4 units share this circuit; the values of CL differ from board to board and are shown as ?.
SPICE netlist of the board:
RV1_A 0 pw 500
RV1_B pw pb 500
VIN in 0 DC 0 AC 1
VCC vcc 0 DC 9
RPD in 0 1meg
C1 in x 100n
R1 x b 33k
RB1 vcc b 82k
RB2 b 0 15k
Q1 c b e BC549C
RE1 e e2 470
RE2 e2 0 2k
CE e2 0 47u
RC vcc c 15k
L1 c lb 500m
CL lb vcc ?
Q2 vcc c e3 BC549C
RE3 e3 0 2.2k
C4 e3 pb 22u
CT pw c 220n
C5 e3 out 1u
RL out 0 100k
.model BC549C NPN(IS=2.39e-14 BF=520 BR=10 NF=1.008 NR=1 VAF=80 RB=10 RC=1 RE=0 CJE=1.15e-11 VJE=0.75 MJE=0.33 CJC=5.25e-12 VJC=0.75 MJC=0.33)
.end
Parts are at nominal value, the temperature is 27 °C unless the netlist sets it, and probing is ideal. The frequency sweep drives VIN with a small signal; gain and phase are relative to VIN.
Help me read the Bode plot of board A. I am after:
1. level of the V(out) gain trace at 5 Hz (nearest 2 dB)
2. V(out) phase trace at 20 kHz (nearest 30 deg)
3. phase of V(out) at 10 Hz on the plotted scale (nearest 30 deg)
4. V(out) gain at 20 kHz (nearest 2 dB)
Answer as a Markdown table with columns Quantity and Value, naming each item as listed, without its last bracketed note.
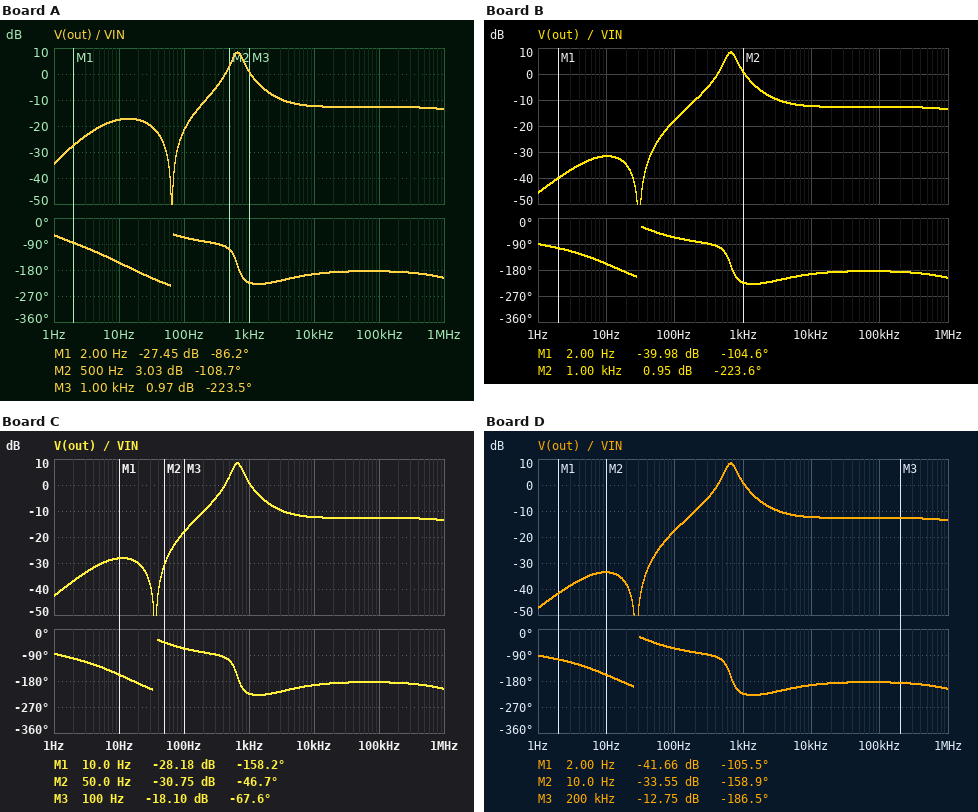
| Quantity | Value |
|---|---|
| level of the V(out) gain trace at 5 Hz | -20 dB |
| V(out) phase trace at 20 kHz | -180 deg |
| phase of V(out) at 10 Hz on the plotted scale | -150 deg |
| V(out) gain at 20 kHz | -12 dB |
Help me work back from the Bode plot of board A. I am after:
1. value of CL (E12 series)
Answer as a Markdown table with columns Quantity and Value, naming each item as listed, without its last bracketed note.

| Quantity | Value |
|---|---|
| value of CL | 12 µF |
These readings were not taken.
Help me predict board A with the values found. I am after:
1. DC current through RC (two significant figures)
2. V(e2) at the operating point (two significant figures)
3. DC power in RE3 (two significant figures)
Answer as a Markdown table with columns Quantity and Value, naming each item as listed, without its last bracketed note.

| Quantity | Value |
|---|---|
| DC current through RC | 320 µA |
| V(e2) at the operating point | 630 mV |
| DC power in RE3 | 5.9 mW |
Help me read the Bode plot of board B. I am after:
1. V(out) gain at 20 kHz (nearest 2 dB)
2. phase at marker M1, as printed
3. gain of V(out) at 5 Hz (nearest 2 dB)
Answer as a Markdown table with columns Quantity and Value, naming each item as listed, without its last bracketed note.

| Quantity | Value |
|---|---|
| V(out) gain at 20 kHz | -12 dB |
| phase at marker M1, as printed | -104.6 deg |
| gain of V(out) at 5 Hz | -34 dB |
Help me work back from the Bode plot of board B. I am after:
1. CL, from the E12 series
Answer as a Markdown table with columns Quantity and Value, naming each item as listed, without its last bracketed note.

| Quantity | Value |
|---|---|
| CL, from the E12 series | 56 µF |
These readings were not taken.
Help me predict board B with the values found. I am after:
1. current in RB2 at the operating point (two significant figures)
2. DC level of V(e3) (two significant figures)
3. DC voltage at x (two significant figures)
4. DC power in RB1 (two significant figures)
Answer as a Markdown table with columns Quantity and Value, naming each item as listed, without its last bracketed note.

| Quantity | Value |
|---|---|
| current in RB2 at the operating point | 92 µA |
| DC level of V(e3) | 3.6 V |
| DC voltage at x | 1.4 V |
| DC power in RB1 | 710 µW |
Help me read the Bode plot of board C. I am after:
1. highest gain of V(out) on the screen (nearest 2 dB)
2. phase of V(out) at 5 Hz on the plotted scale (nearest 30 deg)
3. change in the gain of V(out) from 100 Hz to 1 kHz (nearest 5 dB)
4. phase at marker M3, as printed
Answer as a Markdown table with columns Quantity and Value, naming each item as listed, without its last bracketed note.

| Quantity | Value |
|---|---|
| highest gain of V(out) on the screen | 8 dB |
| phase of V(out) at 5 Hz on the plotted scale | -120 deg |
| change in the gain of V(out) from 100 Hz to 1 kHz | 20 dB |
| phase at marker M3, as printed | -67.6 deg |
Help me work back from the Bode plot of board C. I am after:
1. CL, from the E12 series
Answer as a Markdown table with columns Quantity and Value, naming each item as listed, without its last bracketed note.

| Quantity | Value |
|---|---|
| CL, from the E12 series | 39 µF |
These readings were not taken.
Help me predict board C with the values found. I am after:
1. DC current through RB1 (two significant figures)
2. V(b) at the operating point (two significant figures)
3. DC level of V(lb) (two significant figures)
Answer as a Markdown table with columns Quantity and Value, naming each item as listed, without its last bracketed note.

| Quantity | Value |
|---|---|
| DC current through RB1 | 93 µA |
| V(b) at the operating point | 1.4 V |
| DC level of V(lb) | 4.2 V |
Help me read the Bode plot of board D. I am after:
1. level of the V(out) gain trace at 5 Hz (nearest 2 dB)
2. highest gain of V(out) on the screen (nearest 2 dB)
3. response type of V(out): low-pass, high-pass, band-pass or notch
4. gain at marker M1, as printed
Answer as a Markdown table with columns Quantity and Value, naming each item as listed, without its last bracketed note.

| Quantity | Value |
|---|---|
| level of the V(out) gain trace at 5 Hz | -36 dB |
| highest gain of V(out) on the screen | 8 dB |
| response type of V(out): low-pass, high-pass, band-pass or notch | band-pass |
| gain at marker M1, as printed | -41.66 dB |
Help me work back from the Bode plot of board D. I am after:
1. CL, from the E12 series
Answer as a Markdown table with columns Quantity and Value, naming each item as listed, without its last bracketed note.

| Quantity | Value |
|---|---|
| CL, from the E12 series | 68 µF |
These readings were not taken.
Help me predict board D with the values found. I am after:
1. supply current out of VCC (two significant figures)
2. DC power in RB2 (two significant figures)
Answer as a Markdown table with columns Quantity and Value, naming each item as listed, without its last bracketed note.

| Quantity | Value |
|---|---|
| supply current out of VCC | 2.0 mA |
| DC power in RB2 | 130 µW |
